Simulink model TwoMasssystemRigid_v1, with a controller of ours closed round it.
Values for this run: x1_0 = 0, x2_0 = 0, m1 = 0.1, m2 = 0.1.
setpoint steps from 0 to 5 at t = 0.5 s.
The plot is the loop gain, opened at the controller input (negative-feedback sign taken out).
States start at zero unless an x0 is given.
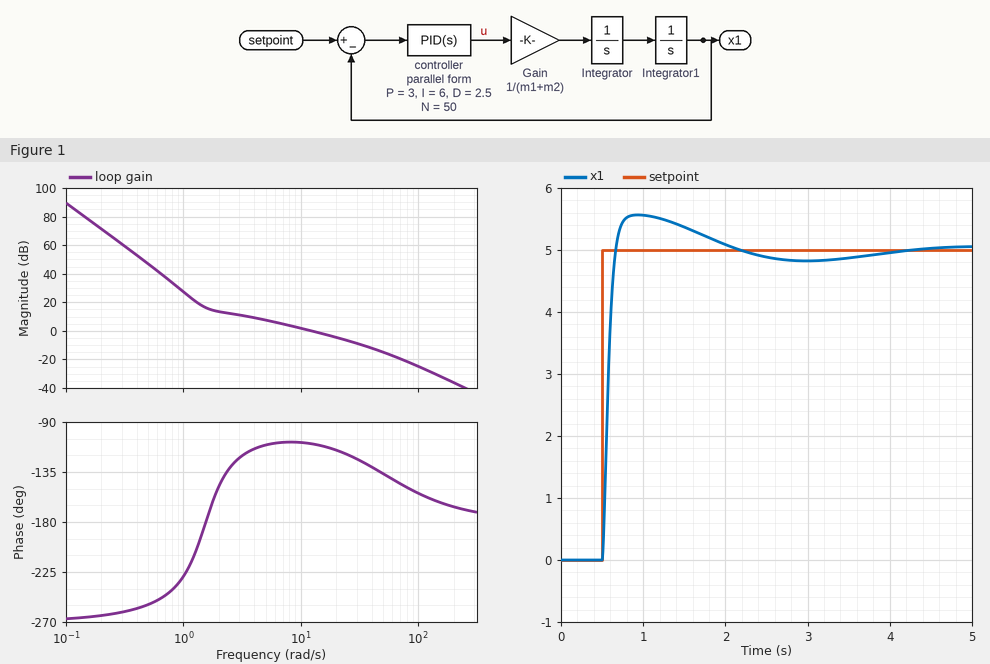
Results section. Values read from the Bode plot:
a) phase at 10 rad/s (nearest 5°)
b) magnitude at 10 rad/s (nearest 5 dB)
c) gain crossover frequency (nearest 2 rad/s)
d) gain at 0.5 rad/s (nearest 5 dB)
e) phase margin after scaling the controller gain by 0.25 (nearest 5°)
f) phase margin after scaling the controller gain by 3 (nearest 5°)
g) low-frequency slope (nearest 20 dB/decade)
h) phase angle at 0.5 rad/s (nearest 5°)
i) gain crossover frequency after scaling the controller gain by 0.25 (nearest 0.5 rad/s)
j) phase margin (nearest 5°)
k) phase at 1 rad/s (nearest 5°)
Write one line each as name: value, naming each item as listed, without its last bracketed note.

phase at 10 rad/s: -110°
magnitude at 10 rad/s: 0 dB
gain crossover frequency: 12 rad/s
gain at 0.5 rad/s: 45 dB
phase margin after scaling the controller gain by 0.25: 50°
phase margin after scaling the controller gain by 3: 55°
low-frequency slope: -60 dB/decade
phase angle at 0.5 rad/s: -255°
gain crossover frequency after scaling the controller gain by 0.25: 2.5 rad/s
phase margin: 70°
phase at 1 rad/s: -230°
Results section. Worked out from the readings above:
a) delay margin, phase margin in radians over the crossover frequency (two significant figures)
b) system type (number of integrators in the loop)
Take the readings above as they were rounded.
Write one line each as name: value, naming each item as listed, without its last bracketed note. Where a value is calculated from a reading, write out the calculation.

delay margin, phase margin in radians over the crossover frequency: 70 × π / 180 / 12 = 0.10 s
system type: 3
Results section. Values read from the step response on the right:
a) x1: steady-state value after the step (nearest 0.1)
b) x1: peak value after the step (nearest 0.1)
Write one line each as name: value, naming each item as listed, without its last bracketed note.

x1: steady-state value after the step: 5.0
x1: peak value after the step: 5.6
